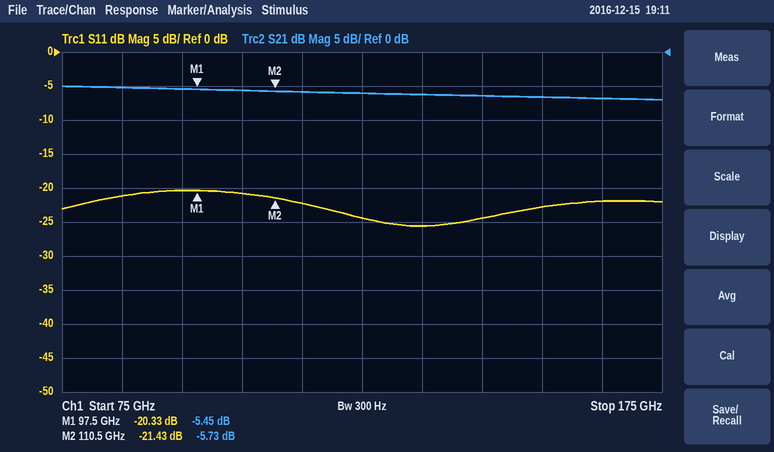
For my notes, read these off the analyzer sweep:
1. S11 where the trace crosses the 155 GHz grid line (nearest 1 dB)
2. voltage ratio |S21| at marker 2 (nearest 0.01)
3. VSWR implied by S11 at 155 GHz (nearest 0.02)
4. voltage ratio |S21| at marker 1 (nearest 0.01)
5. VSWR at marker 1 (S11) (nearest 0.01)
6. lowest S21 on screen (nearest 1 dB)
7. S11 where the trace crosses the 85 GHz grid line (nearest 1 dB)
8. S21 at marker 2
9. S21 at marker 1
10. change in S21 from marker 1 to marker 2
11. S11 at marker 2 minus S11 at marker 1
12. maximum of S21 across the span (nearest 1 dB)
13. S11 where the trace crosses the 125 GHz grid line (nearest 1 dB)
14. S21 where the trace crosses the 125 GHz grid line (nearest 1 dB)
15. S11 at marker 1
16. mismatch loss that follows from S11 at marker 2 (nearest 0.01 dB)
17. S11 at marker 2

-23 dB
0.52
1.16
0.53
1.21
-7 dB
-21 dB
-5.73 dB
-5.45 dB
-0.28 dB
-1.10 dB
-5 dB
-24 dB
-6 dB
-20.33 dB
0.03 dB
-21.43 dB
